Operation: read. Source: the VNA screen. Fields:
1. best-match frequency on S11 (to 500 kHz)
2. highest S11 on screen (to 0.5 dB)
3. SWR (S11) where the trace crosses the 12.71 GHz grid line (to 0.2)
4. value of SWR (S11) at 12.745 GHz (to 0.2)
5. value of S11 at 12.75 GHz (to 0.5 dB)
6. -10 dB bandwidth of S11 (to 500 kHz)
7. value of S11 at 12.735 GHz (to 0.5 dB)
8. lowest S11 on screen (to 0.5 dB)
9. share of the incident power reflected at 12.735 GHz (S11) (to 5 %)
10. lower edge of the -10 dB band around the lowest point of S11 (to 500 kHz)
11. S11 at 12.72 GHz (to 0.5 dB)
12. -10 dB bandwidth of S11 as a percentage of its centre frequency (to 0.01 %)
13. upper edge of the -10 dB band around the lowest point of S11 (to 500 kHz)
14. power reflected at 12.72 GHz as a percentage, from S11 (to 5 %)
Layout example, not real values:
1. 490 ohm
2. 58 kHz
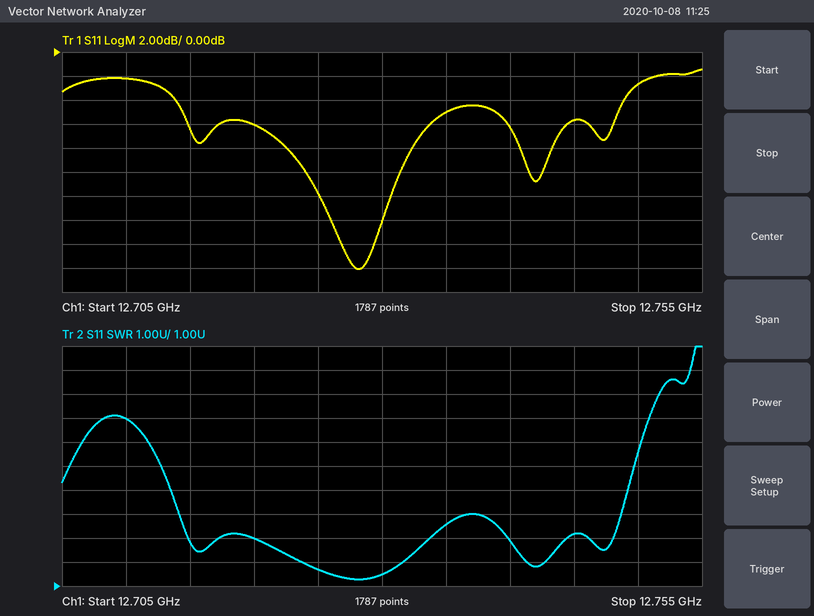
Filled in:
1. 12.7280 GHz
2. -1.5 dB
3. 8.0
4. 3.2
5. -2.5 dB
6. 7.5 MHz
7. -5.0 dB
8. -18.0 dB
9. 30 %
10. 12.7240 GHz
11. -6.0 dB
12. 0.06 %
13. 12.7315 GHz
14. 25 %
